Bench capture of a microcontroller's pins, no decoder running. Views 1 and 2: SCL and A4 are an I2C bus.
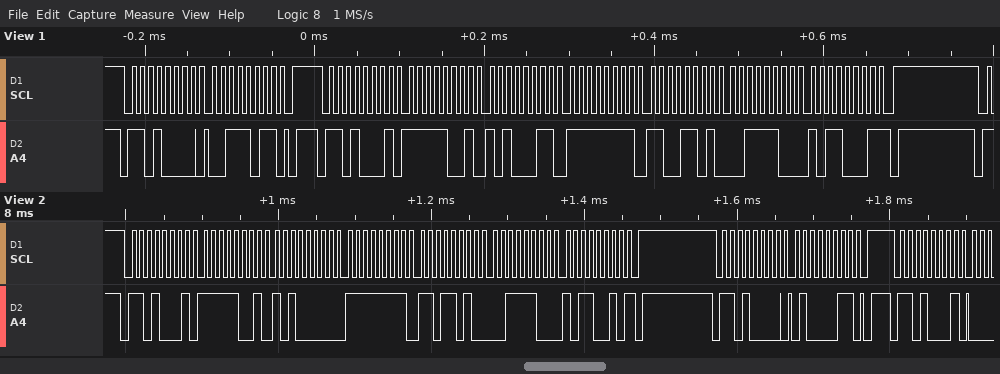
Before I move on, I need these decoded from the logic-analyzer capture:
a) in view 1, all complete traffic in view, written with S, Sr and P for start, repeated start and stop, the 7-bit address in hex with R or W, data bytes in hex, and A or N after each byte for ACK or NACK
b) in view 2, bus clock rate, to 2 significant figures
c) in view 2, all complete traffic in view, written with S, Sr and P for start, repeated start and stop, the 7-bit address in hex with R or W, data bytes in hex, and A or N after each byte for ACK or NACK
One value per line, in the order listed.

S 68W A 3B A P S 68R A F9 A A3 A FF A CD A 3C A B1 N P
100 kHz
S 68R A F9 A A0 A FF A DA A 3C A B2 N P S 68W A 43 A P S 68R A
